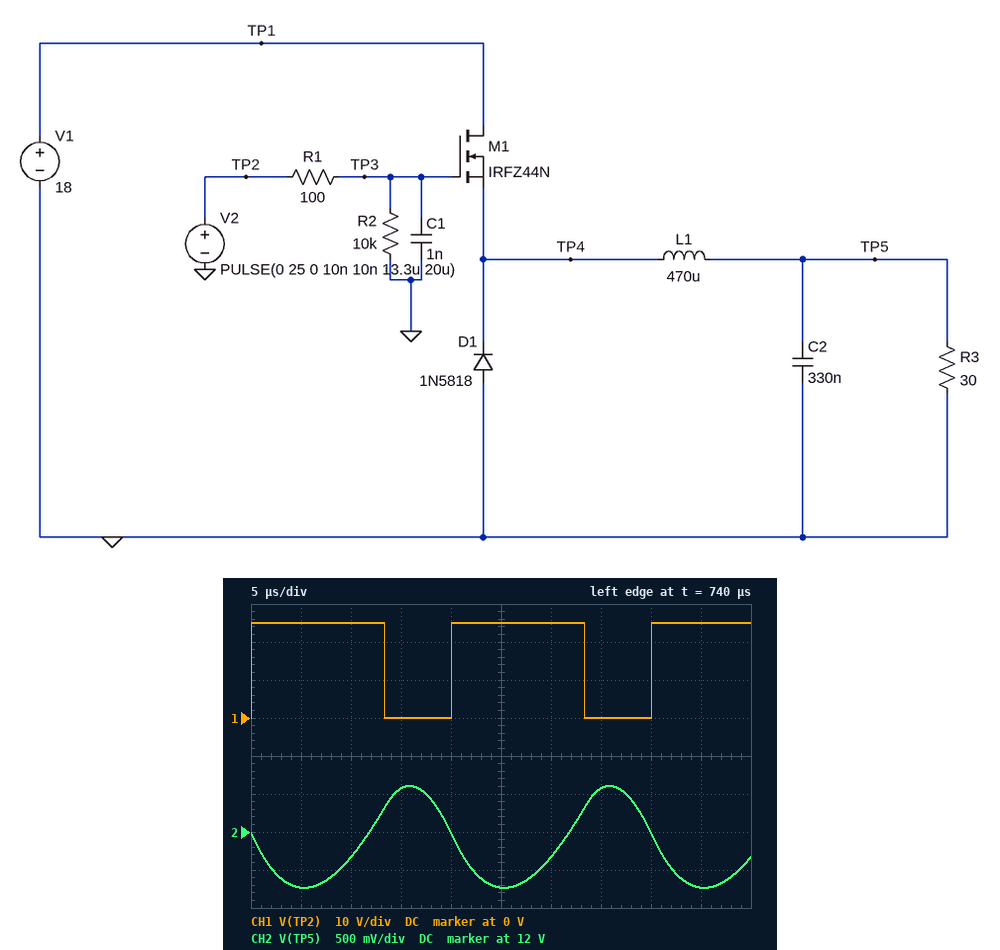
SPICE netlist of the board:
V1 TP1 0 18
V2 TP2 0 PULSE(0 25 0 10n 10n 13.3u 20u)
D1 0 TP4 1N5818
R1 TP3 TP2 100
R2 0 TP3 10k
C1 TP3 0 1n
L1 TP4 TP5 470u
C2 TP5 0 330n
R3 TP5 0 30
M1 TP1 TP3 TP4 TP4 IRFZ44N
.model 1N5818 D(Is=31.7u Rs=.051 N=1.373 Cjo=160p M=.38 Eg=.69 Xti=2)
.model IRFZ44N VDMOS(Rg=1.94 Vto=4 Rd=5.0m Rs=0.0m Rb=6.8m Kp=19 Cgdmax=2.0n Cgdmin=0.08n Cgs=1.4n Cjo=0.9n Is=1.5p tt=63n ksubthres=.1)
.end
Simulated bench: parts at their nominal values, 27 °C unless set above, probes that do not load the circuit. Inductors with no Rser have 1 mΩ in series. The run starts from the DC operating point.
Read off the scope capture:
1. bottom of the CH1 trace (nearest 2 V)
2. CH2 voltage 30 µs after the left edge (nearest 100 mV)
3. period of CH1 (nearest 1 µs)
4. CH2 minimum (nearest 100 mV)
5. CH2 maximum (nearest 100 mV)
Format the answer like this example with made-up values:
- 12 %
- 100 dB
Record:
- 0 V
- 11.7 V
- 20 µs
- 11.3 V
- 12.6 V
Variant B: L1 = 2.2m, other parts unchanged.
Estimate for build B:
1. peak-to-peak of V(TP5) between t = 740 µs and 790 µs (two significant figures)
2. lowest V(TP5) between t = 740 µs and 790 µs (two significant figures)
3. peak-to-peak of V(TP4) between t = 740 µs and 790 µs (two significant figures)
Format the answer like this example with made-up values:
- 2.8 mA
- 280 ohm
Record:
- 270 mV
- 12 V
- 18 V
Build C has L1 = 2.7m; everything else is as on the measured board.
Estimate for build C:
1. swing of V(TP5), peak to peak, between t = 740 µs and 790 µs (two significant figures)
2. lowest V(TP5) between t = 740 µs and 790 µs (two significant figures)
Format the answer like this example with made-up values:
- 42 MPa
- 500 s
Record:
- 220 mV
- 12 V
